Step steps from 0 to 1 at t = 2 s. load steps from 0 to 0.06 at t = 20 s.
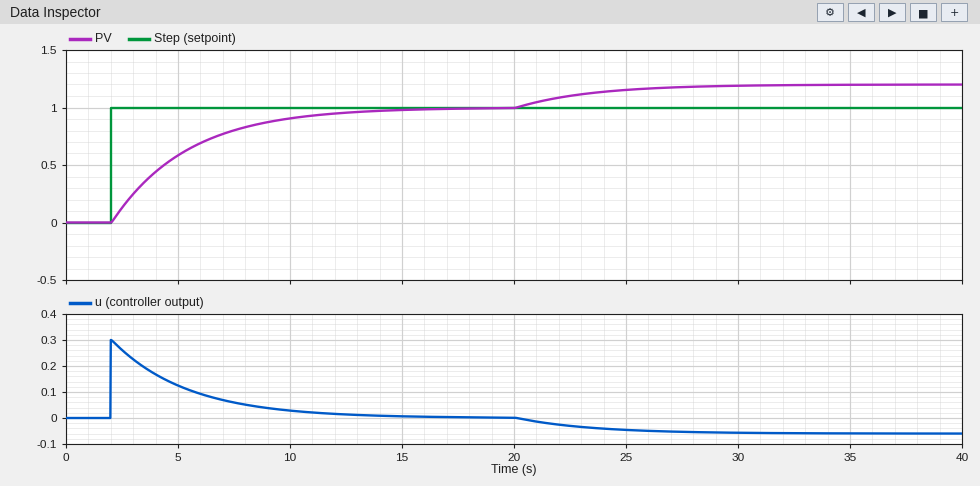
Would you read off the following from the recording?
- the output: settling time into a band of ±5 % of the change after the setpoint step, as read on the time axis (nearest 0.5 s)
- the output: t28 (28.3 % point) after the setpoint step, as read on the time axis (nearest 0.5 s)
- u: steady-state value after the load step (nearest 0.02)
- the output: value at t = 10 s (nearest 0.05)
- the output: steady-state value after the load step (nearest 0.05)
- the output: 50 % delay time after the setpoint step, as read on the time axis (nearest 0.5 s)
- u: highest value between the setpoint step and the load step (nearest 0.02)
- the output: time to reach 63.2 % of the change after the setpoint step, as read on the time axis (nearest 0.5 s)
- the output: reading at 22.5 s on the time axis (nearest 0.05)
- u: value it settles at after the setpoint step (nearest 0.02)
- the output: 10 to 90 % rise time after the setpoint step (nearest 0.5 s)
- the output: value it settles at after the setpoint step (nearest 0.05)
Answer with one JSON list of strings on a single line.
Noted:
["12.0 s", "3.0 s", "-0.06", "0.90", "1.20", "4.5 s", "0.30", "5.5 s", "1.10", "0.00", "7.5 s", "1.00"]
